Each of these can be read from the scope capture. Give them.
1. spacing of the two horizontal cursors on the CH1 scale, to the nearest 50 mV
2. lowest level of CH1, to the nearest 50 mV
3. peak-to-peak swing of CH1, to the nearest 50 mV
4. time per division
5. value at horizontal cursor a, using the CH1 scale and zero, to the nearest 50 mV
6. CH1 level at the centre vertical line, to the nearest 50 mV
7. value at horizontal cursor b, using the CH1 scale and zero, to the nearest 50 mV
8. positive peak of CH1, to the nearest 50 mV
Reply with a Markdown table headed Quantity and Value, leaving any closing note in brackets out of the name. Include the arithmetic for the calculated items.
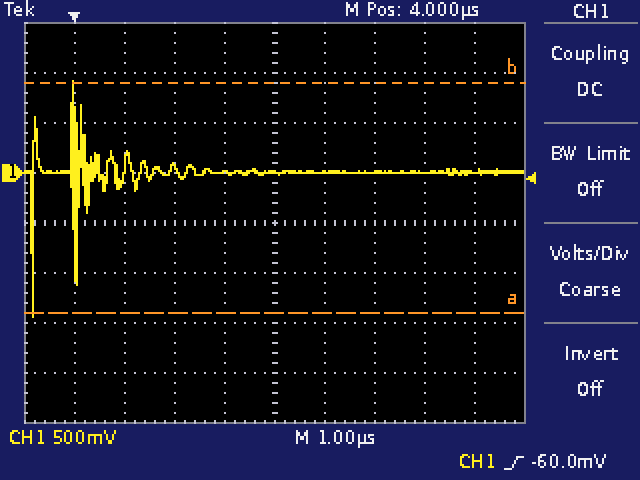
| Quantity | Value |
|---|---|
| spacing of the two horizontal cursors on the CH1 scale, to the nearest 50 mV | 2.30 V |
| lowest level of CH1, to the nearest 50 mV | -1.45 V |
| peak-to-peak swing of CH1, to the nearest 50 mV | 900 mV − (-1.45 V) = 2.35 V |
| time per division | 1 µs |
| value at horizontal cursor a, using the CH1 scale and zero, to the nearest 50 mV | -1.40 V |
| CH1 level at the centre vertical line, to the nearest 50 mV | 0 mV |
| value at horizontal cursor b, using the CH1 scale and zero, to the nearest 50 mV | 900 mV |
| positive peak of CH1, to the nearest 50 mV | 900 mV |
